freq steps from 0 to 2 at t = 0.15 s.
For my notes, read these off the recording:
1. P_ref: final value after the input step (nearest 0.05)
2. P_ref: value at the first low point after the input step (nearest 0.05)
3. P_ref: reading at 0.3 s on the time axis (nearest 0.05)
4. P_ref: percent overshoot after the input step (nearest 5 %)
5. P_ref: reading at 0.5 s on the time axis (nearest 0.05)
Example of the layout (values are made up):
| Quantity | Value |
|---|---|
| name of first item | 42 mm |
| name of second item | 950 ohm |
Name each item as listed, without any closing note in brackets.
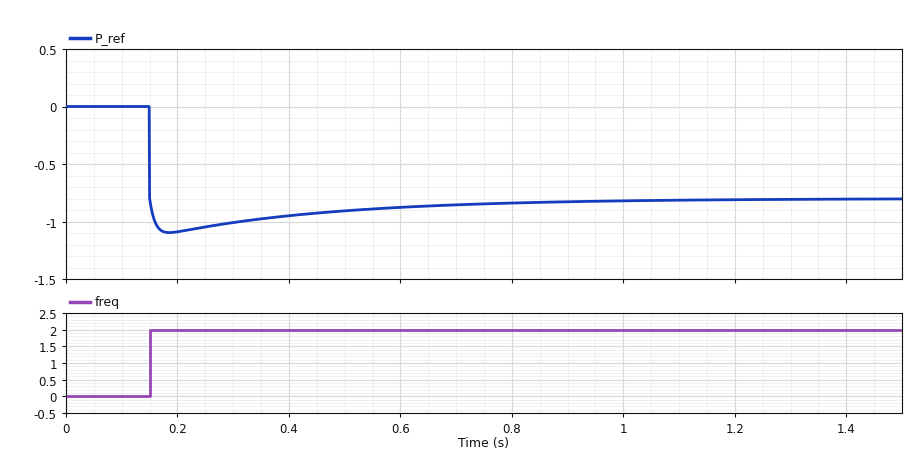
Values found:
| Quantity | Value |
|---|---|
| P_ref: final value after the input step | -0.80 |
| P_ref: value at the first low point after the input step | -1.10 |
| P_ref: reading at 0.3 s on the time axis | -1.00 |
| P_ref: percent overshoot after the input step | 35 % |
| P_ref: reading at 0.5 s on the time axis | -0.90 |
